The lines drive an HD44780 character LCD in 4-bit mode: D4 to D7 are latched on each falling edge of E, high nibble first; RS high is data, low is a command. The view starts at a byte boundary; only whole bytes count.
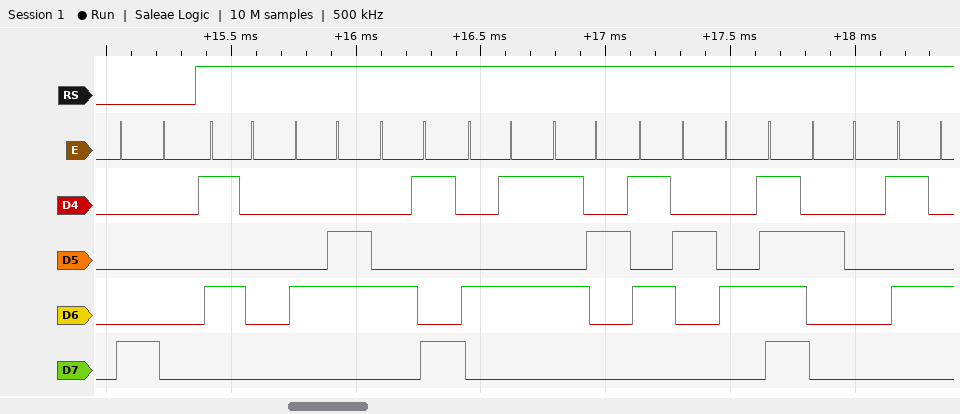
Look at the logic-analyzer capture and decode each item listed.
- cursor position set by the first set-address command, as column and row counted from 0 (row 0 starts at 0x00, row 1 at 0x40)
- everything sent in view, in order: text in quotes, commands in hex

column 0, row 0
0x80 "PFIERRO T"
